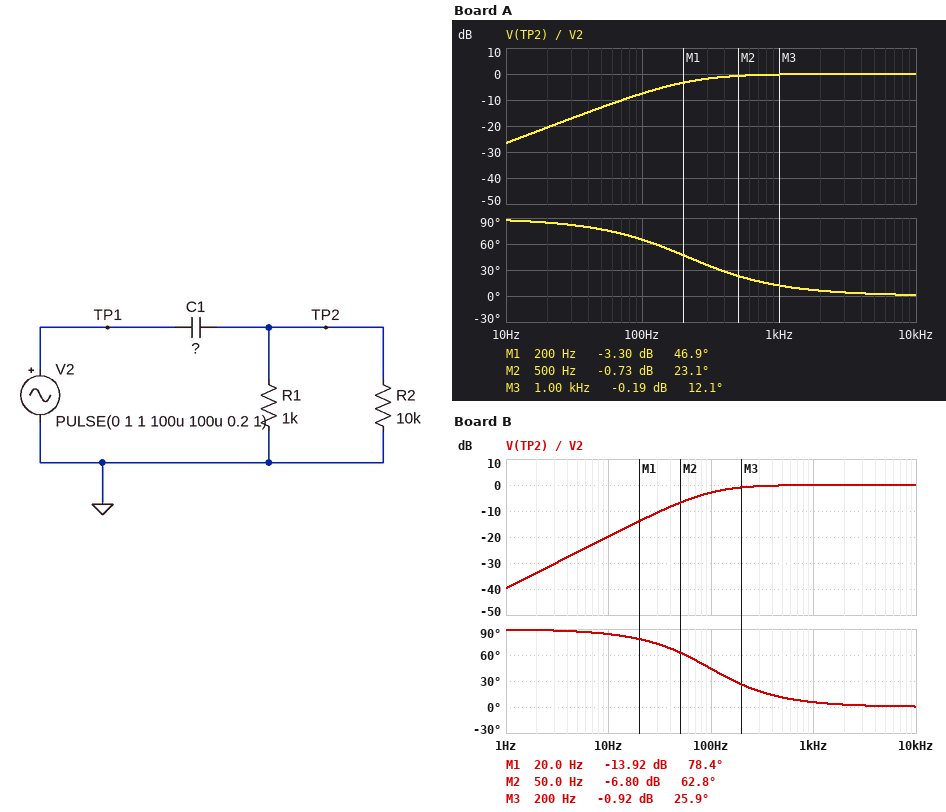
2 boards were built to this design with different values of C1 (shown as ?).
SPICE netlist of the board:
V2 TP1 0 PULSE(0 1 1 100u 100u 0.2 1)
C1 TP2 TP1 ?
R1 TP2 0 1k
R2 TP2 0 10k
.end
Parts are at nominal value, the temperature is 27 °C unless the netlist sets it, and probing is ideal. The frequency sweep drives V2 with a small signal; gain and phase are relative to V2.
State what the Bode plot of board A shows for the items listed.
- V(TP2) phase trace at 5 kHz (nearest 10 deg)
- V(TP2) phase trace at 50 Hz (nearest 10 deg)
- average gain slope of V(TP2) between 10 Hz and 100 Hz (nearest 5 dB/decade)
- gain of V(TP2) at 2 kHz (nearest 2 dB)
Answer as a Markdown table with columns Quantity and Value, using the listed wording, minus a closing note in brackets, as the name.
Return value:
| Quantity | Value |
|---|---|
| V(TP2) phase trace at 5 kHz | 0 deg |
| V(TP2) phase trace at 50 Hz | 80 deg |
| average gain slope of V(TP2) between 10 Hz and 100 Hz | 20 dB/decade |
| gain of V(TP2) at 2 kHz | 0 dB |
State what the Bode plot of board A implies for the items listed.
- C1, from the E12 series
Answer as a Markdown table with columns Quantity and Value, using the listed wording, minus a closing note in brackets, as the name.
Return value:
| Quantity | Value |
|---|---|
| C1, from the E12 series | 820 nF |
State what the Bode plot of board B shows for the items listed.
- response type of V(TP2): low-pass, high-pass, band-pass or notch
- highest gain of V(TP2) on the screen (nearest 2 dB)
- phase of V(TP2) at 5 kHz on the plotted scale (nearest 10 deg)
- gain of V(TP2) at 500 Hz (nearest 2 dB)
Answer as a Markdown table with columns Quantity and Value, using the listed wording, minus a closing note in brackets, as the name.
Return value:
| Quantity | Value |
|---|---|
| response type of V(TP2): low-pass, high-pass, band-pass or notch | high-pass |
| highest gain of V(TP2) on the screen | 0 dB |
| phase of V(TP2) at 5 kHz on the plotted scale | 0 deg |
| gain of V(TP2) at 500 Hz | 0 dB |
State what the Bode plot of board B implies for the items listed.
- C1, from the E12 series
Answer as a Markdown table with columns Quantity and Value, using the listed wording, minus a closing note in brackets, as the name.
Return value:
| Quantity | Value |
|---|---|
| C1, from the E12 series | 1.8 µF |
